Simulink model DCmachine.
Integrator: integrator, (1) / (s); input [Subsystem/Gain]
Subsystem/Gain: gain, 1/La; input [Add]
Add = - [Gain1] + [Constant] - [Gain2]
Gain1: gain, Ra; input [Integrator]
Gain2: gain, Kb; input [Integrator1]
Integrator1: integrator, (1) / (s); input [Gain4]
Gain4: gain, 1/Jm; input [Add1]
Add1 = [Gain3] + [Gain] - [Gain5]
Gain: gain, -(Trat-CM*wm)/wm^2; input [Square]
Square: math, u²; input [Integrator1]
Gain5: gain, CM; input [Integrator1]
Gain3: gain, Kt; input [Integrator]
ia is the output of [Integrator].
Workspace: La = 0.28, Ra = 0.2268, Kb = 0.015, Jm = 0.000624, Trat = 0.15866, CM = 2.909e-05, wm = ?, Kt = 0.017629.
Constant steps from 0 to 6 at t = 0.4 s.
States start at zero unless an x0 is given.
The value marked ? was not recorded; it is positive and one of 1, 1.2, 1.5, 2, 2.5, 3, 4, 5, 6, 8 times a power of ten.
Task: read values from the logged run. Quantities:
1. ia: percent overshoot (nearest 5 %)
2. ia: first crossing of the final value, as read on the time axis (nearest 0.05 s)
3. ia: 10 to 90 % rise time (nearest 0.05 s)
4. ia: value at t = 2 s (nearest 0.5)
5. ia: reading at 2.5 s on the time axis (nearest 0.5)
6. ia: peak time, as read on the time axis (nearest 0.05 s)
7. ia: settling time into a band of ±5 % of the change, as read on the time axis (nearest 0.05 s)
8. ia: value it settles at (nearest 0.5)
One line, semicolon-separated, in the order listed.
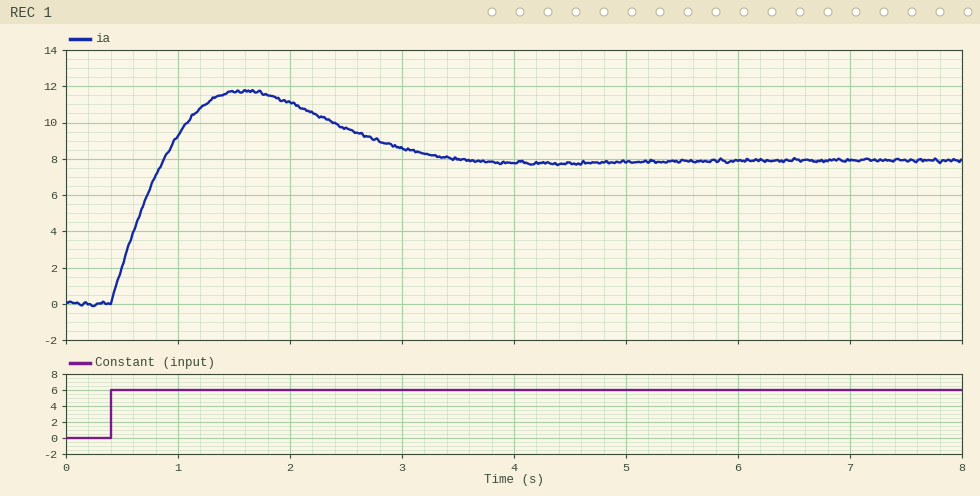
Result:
50 %; 0.85 s; 0.35 s; 11.0; 9.5; 1.60 s; 3.20 s; 8.0
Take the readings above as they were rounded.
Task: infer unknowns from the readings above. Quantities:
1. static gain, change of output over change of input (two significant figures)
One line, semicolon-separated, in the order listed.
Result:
1.3
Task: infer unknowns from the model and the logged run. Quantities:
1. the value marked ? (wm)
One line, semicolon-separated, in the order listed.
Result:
300
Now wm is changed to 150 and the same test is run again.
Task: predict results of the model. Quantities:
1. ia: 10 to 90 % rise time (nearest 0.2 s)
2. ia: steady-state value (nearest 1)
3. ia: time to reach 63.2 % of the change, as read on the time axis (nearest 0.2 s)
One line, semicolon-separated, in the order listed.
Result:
1.2 s; 14; 1.0 s
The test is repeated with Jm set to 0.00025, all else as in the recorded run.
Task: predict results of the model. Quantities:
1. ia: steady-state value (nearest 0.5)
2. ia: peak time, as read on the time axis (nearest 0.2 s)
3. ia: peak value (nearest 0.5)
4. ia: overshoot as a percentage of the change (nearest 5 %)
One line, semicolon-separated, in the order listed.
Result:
8.0; 1.4 s; 9.0; 15 %
